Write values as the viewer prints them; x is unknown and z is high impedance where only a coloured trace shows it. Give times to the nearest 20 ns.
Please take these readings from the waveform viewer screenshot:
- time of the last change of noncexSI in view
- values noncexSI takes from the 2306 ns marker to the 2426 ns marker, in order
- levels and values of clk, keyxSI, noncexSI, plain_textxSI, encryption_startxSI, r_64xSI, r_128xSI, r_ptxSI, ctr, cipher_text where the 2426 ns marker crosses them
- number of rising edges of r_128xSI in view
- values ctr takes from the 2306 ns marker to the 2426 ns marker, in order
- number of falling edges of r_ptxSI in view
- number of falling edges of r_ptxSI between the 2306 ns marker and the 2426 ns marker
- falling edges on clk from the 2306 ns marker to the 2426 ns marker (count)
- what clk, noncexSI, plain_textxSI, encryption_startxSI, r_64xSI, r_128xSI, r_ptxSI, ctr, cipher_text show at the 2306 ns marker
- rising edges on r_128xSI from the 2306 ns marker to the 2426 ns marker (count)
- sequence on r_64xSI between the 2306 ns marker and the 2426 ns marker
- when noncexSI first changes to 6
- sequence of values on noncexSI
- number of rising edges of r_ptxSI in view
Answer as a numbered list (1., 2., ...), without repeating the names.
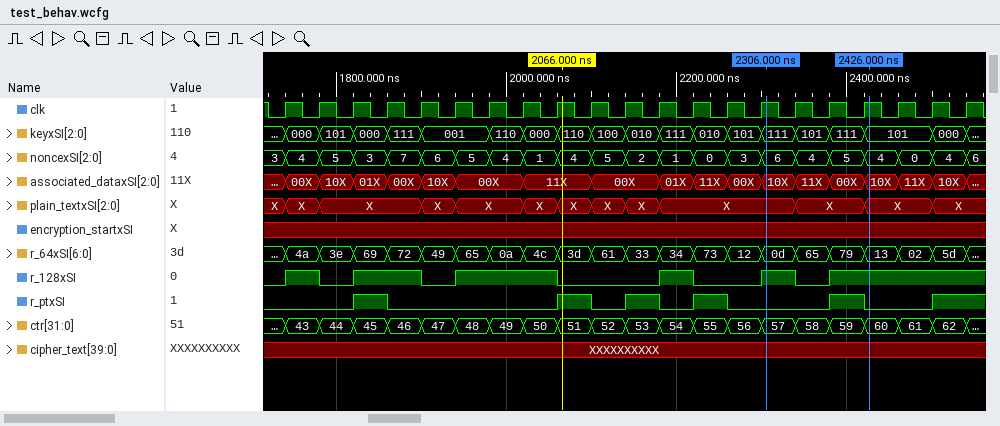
1. 2540 ns
2. 6, 4, 5, 4
3. clk=1, keyxSI=101, noncexSI=4, plain_textxSI=X, encryption_startxSI=x, r_64xSI=13, r_128xSI=1, r_ptxSI=0, ctr=60, cipher_text=XXXXXXXXXX
4. 6
5. 57, 58, 59, 60
6. 5
7. 1
8. 3
9. clk=1, noncexSI=6, plain_textxSI=X, encryption_startxSI=x, r_64xSI=0d, r_128xSI=1, r_ptxSI=0, ctr=57, cipher_text=XXXXXXXXXX
10. 1
11. 0d, 65, 79, 13
12. 1900 ns
13. 3, 4, 5, 3, 7, 6, 5, 4, 1, 4, 5, 2, 1, 0, 3, 6, 4, 5, 4, 0, 4, 6
14. 6
